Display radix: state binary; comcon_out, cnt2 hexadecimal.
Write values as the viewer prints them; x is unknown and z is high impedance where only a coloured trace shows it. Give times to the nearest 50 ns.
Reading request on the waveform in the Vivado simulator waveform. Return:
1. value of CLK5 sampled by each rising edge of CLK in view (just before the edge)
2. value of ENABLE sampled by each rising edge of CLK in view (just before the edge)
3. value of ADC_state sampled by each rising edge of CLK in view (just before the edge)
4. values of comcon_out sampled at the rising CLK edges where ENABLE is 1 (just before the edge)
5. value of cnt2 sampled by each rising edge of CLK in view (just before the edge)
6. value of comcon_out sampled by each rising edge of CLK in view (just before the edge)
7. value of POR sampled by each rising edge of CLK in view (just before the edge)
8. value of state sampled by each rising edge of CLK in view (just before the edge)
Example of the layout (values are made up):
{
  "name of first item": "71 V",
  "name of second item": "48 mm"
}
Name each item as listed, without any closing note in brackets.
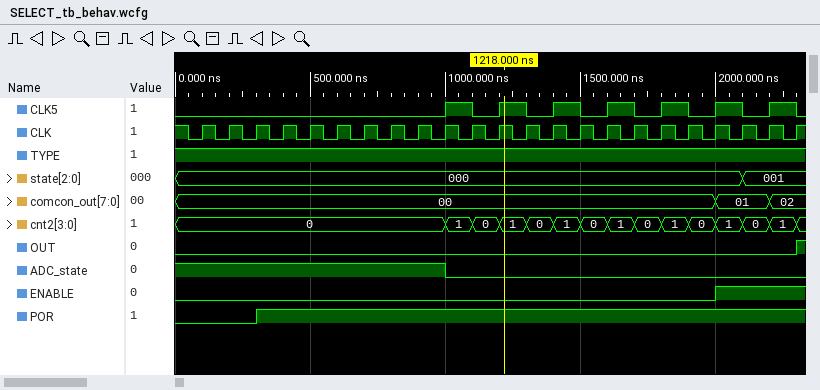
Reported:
{
  "value of CLK5 sampled by each rising edge of CLK in view": "0 0 0 0 0 0 0 0 0 0 1 0 1 0 1 0 1 0 1 0 1 0 1",
  "value of ENABLE sampled by each rising edge of CLK in view": "0 0 0 0 0 0 0 0 0 0 0 0 0 0 0 0 0 0 0 0 1 1 1",
  "value of ADC_state sampled by each rising edge of CLK in view": "1 1 1 1 1 1 1 1 1 1 0 0 0 0 0 0 0 0 0 0 0 0 0",
  "values of comcon_out sampled at the rising CLK edges where ENABLE is 1": "01, 01, 02",
  "value of cnt2 sampled by each rising edge of CLK in view": "0, 0, 0, 0, 0, 0, 0, 0, 0, 0, 1, 0, 1, 0, 1, 0, 1, 0, 1, 0, 1, 0, 1",
  "value of comcon_out sampled by each rising edge of CLK in view": "00, 00, 00, 00, 00, 00, 00, 00, 00, 00, 00, 00, 00, 00, 00, 00, 00, 00, 00, 00, 01, 01, 02",
  "value of POR sampled by each rising edge of CLK in view": "0 0 0 1 1 1 1 1 1 1 1 1 1 1 1 1 1 1 1 1 1 1 1",
  "value of state sampled by each rising edge of CLK in view": "000, 000, 000, 000, 000, 000, 000, 000, 000, 000, 000, 000, 000, 000, 000, 000, 000, 000, 000, 000, 000, 001, 001"
}
